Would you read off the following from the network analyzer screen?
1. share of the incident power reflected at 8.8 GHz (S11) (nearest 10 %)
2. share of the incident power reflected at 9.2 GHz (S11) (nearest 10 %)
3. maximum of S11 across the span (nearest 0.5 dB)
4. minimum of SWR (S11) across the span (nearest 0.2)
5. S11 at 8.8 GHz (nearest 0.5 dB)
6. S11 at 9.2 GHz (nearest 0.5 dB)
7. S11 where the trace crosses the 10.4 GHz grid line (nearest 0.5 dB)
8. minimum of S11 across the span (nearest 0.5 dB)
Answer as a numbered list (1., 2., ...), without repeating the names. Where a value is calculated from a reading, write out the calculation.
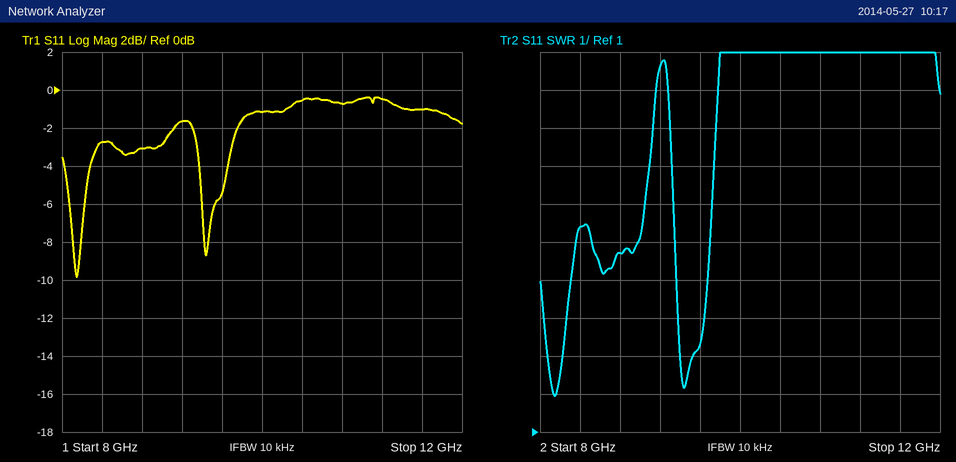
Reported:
1. 10^(-3/10) ≈ 50 %
2. 10^(-1.5/10) ≈ 70.8 %, so 70 % to the nearest 10 %
3. -0.5 dB
4. 2.0
5. -3.0 dB
6. -1.5 dB
7. -0.5 dB
8. -10.0 dB
